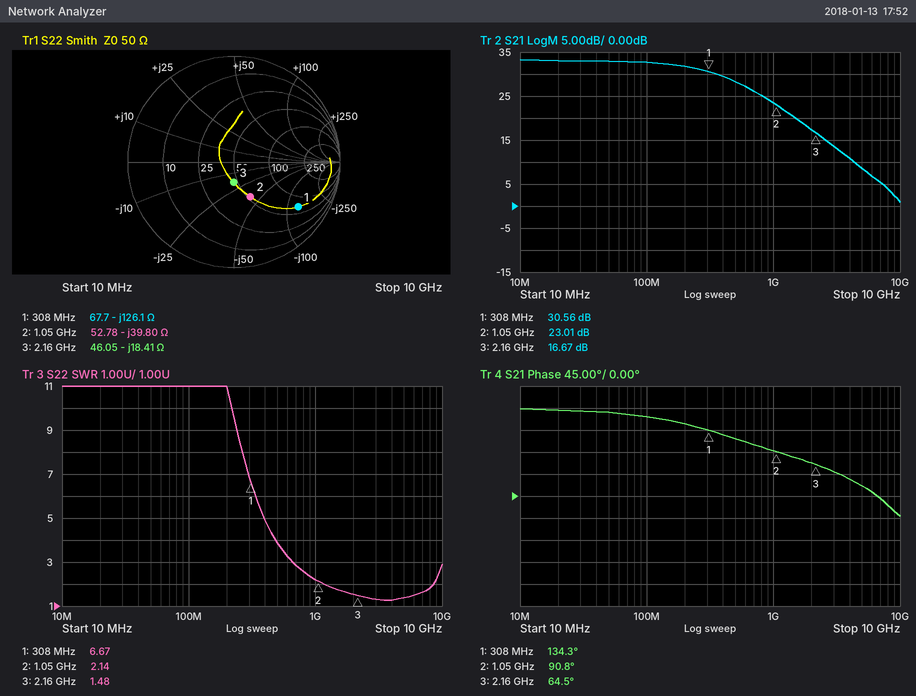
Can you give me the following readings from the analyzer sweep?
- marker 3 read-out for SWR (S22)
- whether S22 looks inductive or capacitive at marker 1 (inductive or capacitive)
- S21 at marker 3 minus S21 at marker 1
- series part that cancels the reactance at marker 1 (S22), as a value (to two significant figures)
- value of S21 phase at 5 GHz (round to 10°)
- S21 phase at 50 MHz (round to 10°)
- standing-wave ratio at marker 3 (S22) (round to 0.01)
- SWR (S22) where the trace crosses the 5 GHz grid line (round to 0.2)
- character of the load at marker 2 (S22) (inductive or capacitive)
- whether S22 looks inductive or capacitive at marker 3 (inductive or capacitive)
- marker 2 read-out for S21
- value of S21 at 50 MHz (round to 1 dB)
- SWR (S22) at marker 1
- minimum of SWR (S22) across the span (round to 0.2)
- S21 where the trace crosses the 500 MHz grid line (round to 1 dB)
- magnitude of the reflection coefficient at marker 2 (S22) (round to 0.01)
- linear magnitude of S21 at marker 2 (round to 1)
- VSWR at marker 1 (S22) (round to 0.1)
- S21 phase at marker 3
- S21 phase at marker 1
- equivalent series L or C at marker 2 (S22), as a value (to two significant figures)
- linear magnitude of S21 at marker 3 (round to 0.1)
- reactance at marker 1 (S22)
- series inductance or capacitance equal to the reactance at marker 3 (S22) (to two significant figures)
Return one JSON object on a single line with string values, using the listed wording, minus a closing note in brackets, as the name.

{"marker 3 read-out for SWR": "1.48", "whether S22 looks inductive or capacitive at marker 1": "capacitive", "S21 at marker 3 minus S21 at marker 1": "-13.89 dB", "series part that cancels the reactance at marker 1 (S22), as a value": "65 nH", "value of S21 phase at 5 GHz": "20°", "S21 phase at 50 MHz": "170°", "standing-wave ratio at marker 3 (S22)": "1.48", "SWR (S22) where the trace crosses the 5 GHz grid line": "1.4", "character of the load at marker 2 (S22)": "capacitive", "whether S22 looks inductive or capacitive at marker 3": "capacitive", "marker 2 read-out for S21": "23.01 dB", "value of S21 at 50 MHz": "33 dB", "SWR (S22) at marker 1": "6.67", "minimum of SWR (S22) across the span": "1.2", "S21 where the trace crosses the 500 MHz grid line": "28 dB", "magnitude of the reflection coefficient at marker 2 (S22)": "0.36", "linear magnitude of S21 at marker 2": "14", "VSWR at marker 1 (S22)": "6.6", "S21 phase at marker 3": "64.5°", "S21 phase at marker 1": "134.3°", "equivalent series L or C at marker 2 (S22), as a value": "3.8 pF", "linear magnitude of S21 at marker 3": "6.8", "reactance at marker 1": "-126.1 Ω", "series inductance or capacitance equal to the reactance at marker 3 (S22)": "4.0 pF"}
